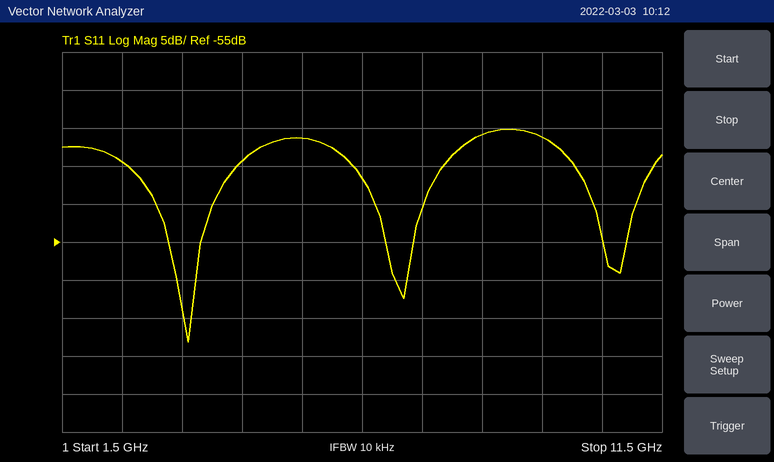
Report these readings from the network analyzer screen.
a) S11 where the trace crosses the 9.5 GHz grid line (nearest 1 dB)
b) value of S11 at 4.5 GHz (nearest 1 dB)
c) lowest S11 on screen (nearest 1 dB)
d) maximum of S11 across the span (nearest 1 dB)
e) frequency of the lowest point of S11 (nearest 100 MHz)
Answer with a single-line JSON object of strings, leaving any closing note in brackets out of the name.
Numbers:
{"S11 where the trace crosses the 9.5 GHz grid line": "-41 dB", "value of S11 at 4.5 GHz": "-44 dB", "lowest S11 on screen": "-68 dB", "maximum of S11 across the span": "-40 dB", "frequency of the lowest point of S11": "3.6 GHz"}
